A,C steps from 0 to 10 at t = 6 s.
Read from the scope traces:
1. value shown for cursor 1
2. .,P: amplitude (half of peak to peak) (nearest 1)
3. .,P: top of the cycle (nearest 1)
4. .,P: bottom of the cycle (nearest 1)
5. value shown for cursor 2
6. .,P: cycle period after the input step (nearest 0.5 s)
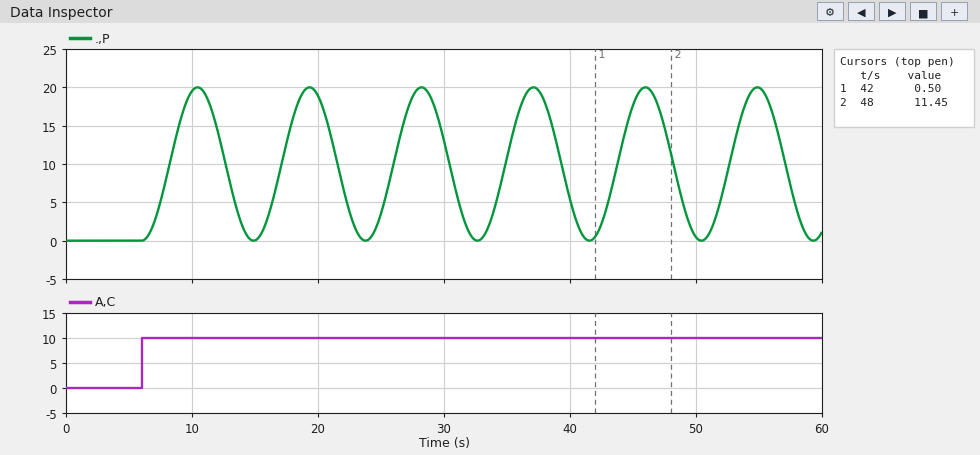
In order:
0.50
10
20
0
11.45
9.0 s
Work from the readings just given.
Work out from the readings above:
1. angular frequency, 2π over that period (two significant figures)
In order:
0.70 rad/s
